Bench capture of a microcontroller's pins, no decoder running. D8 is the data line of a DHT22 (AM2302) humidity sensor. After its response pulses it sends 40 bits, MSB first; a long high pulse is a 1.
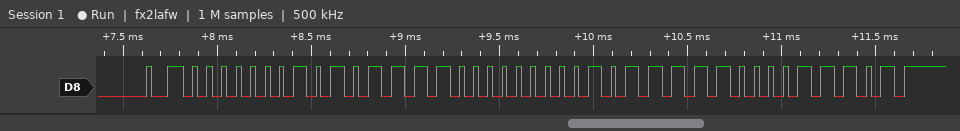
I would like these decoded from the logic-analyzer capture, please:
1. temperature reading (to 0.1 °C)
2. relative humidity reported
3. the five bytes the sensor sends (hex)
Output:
19.0 °C
35.0 %
01 5E 00 BE 1D
